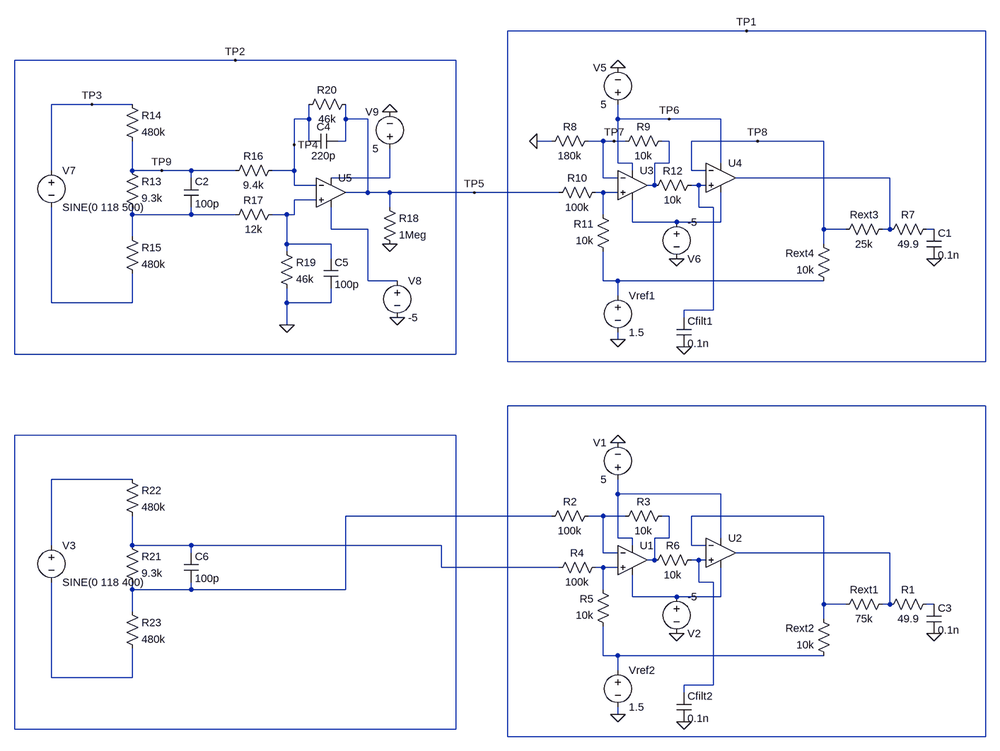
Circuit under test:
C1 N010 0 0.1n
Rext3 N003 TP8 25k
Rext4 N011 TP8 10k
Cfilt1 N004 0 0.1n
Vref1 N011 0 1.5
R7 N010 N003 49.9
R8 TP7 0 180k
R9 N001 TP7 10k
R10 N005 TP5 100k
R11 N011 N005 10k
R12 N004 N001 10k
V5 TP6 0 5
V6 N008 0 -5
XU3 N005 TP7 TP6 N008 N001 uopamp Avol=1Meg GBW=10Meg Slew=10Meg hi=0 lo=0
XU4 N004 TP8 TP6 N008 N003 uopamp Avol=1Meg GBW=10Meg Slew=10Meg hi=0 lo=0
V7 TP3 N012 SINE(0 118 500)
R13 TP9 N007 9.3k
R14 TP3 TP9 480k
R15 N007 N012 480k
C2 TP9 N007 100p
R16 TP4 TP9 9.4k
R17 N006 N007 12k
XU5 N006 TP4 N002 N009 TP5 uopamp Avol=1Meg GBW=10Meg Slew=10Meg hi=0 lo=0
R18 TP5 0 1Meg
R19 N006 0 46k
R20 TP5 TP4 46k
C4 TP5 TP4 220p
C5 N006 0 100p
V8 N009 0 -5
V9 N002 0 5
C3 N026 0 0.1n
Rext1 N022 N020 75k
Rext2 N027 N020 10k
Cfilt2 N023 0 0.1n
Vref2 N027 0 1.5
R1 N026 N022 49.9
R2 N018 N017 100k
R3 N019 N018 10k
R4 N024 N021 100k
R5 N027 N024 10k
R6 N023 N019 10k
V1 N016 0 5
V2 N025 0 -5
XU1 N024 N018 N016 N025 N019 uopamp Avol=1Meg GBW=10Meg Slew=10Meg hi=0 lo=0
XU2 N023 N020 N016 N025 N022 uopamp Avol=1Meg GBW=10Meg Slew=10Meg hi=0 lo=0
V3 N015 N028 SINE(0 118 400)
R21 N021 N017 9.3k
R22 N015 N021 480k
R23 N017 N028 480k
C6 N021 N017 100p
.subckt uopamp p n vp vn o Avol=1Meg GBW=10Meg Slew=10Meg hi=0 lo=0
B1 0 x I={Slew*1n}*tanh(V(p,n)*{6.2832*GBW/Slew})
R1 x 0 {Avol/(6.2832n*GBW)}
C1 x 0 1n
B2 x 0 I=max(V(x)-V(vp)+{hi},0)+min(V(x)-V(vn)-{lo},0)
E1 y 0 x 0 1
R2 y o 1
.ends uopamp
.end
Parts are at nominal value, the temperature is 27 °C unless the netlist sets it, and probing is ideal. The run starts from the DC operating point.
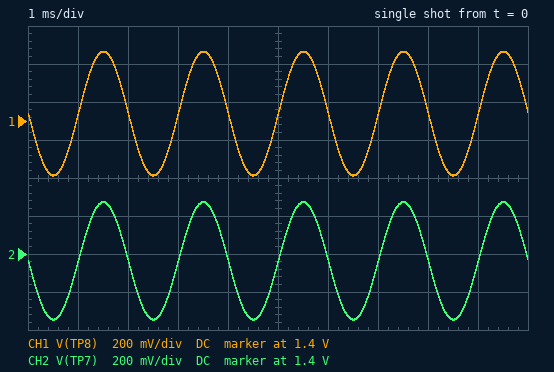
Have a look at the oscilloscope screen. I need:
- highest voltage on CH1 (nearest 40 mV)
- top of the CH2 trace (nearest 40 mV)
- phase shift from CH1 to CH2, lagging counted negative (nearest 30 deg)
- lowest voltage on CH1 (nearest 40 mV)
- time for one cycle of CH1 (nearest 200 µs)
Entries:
1.76 V
1.68 V
0 deg
1.12 V
2.0 ms
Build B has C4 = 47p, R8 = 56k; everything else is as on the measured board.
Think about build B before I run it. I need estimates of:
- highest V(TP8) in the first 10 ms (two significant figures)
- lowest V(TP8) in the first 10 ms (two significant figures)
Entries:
2.0 V
1.2 V
